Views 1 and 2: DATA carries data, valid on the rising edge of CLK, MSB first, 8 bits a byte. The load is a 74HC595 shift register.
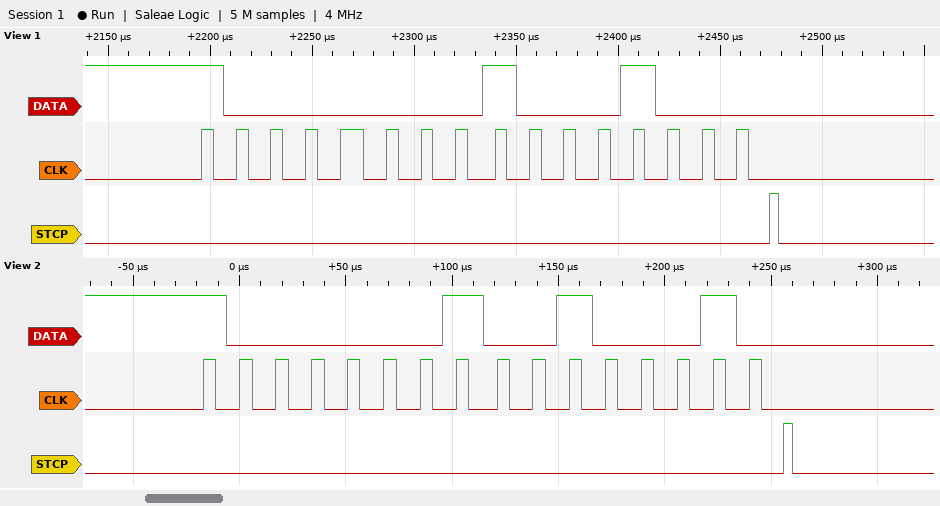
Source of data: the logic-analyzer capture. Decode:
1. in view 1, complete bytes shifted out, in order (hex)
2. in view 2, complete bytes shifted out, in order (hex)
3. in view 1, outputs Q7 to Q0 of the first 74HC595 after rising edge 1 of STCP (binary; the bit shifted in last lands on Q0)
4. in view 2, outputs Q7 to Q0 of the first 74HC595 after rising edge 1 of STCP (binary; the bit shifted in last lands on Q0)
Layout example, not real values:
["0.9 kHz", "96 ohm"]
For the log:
["80 88", "81 22", "10001000", "00100010"]
